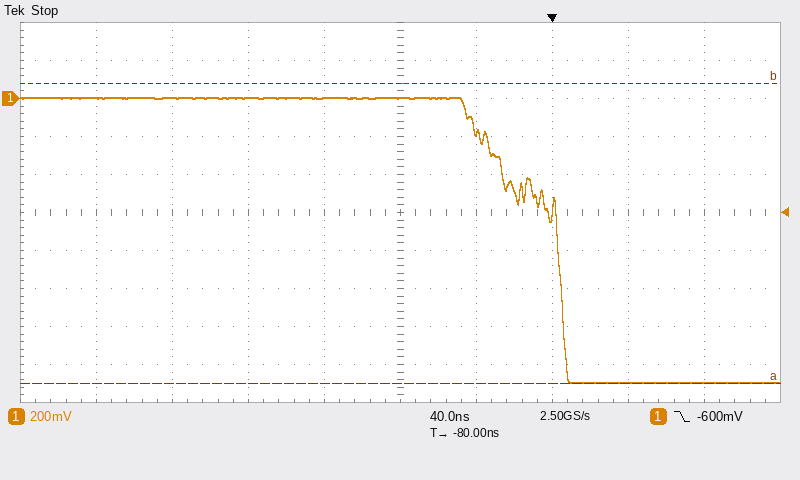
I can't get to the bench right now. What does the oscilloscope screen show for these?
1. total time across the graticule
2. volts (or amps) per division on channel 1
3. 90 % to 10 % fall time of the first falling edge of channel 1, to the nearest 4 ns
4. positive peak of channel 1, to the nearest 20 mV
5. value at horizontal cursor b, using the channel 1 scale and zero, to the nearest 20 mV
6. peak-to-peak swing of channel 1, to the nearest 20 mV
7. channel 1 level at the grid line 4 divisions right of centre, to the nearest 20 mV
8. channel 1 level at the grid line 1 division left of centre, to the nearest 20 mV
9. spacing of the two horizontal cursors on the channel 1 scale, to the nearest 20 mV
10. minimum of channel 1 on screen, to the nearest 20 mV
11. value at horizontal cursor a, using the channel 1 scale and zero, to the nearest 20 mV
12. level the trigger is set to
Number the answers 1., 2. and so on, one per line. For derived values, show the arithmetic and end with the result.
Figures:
1. 400 ns
2. 200 mV
3. 48 ns
4. 0 mV
5. 80 mV
6. 0 mV − (-1.50 V) = 1.50 V
7. -1.50 V
8. 0 mV
9. 1.58 V
10. -1.50 V
11. -1.50 V
12. -600 mV
